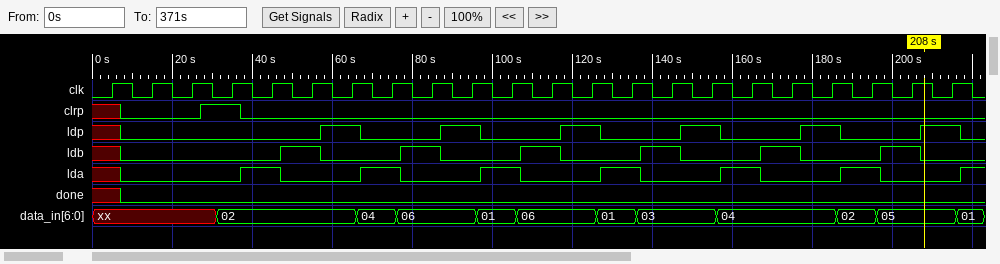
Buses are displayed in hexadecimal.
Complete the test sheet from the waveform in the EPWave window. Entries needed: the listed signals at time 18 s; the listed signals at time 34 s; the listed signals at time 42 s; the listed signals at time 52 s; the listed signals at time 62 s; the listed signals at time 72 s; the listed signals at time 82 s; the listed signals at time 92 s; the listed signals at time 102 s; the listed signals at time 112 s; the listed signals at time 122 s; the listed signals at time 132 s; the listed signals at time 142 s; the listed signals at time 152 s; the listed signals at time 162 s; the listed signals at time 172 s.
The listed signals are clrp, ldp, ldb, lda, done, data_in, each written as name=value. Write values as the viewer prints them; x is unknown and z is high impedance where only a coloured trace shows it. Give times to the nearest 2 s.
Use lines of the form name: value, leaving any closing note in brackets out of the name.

the listed signals at time 18 s: clrp=0, ldp=0, ldb=0, lda=0, done=0, data_in=xx
the listed signals at time 34 s: clrp=1, ldp=0, ldb=0, lda=0, done=0, data_in=02
the listed signals at time 42 s: clrp=0, ldp=0, ldb=0, lda=1, done=0, data_in=02
the listed signals at time 52 s: clrp=0, ldp=0, ldb=1, lda=0, done=0, data_in=02
the listed signals at time 62 s: clrp=0, ldp=1, ldb=0, lda=0, done=0, data_in=02
the listed signals at time 72 s: clrp=0, ldp=0, ldb=0, lda=1, done=0, data_in=04
the listed signals at time 82 s: clrp=0, ldp=0, ldb=1, lda=0, done=0, data_in=06
the listed signals at time 92 s: clrp=0, ldp=1, ldb=0, lda=0, done=0, data_in=06
the listed signals at time 102 s: clrp=0, ldp=0, ldb=0, lda=1, done=0, data_in=01
the listed signals at time 112 s: clrp=0, ldp=0, ldb=1, lda=0, done=0, data_in=06
the listed signals at time 122 s: clrp=0, ldp=1, ldb=0, lda=0, done=0, data_in=06
the listed signals at time 132 s: clrp=0, ldp=0, ldb=0, lda=1, done=0, data_in=01
the listed signals at time 142 s: clrp=0, ldp=0, ldb=1, lda=0, done=0, data_in=03
the listed signals at time 152 s: clrp=0, ldp=1, ldb=0, lda=0, done=0, data_in=03
the listed signals at time 162 s: clrp=0, ldp=0, ldb=0, lda=1, done=0, data_in=04
the listed signals at time 172 s: clrp=0, ldp=0, ldb=1, lda=0, done=0, data_in=04
